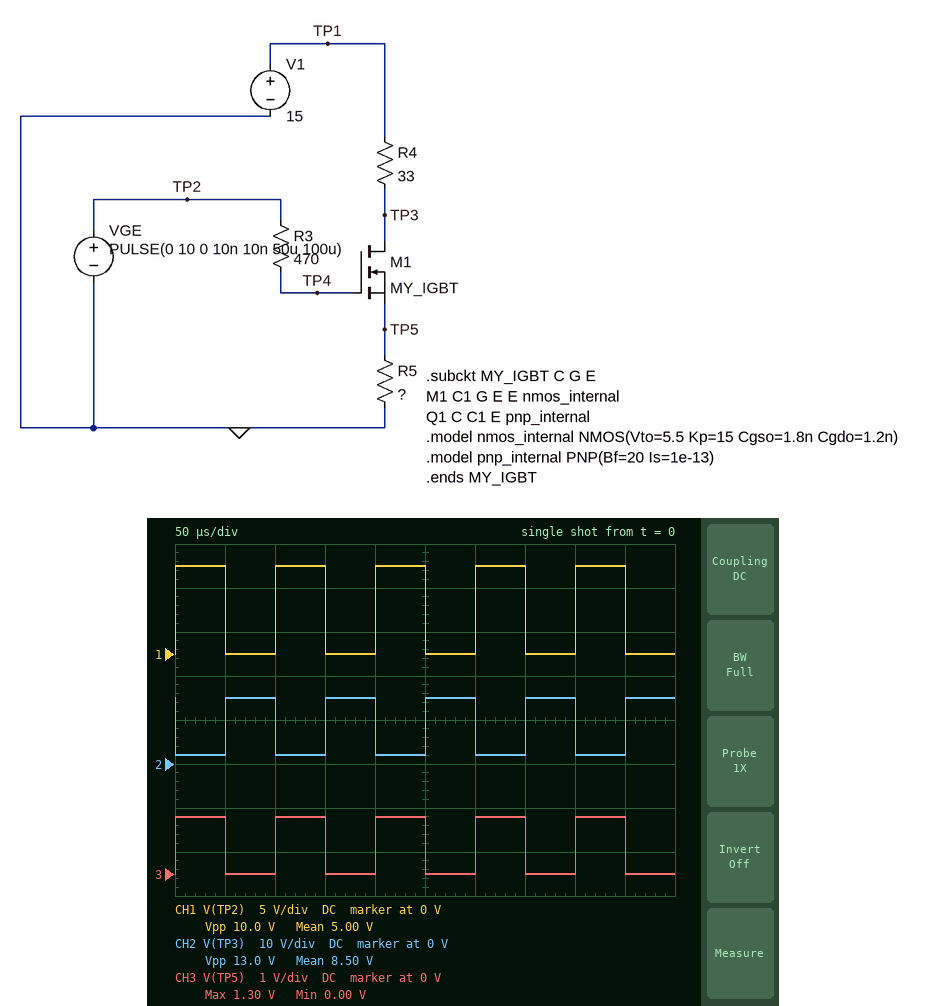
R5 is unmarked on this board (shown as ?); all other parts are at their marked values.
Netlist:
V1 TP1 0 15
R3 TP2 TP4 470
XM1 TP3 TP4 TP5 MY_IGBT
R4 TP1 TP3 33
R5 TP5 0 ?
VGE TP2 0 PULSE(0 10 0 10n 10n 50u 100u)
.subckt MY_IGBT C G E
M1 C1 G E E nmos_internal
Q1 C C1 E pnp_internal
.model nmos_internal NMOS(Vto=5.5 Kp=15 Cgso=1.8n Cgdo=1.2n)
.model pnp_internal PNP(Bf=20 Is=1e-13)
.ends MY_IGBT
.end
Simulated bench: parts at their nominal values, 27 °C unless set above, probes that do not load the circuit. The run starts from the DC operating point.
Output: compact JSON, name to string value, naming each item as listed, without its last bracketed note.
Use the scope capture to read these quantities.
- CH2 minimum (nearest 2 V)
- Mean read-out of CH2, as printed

{"CH2 minimum": "2 V", "Mean read-out of CH2, as printed": "8.50 V"}
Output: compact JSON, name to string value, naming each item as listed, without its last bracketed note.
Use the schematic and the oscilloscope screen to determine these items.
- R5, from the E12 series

{"R5, from the E12 series": "3.3 Ω"}
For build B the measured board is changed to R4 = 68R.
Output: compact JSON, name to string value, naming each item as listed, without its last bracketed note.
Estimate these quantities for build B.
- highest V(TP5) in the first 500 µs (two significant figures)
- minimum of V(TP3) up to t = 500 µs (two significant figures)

{"highest V(TP5) in the first 500 µs": "670 mV", "minimum of V(TP3) up to t = 500 µs": "1.4 V"}
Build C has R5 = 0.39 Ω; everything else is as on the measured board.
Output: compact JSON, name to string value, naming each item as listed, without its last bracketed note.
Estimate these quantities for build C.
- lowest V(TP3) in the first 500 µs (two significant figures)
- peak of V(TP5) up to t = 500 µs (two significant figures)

{"lowest V(TP3) in the first 500 µs": "900 mV", "peak of V(TP5) up to t = 500 µs": "170 mV"}
